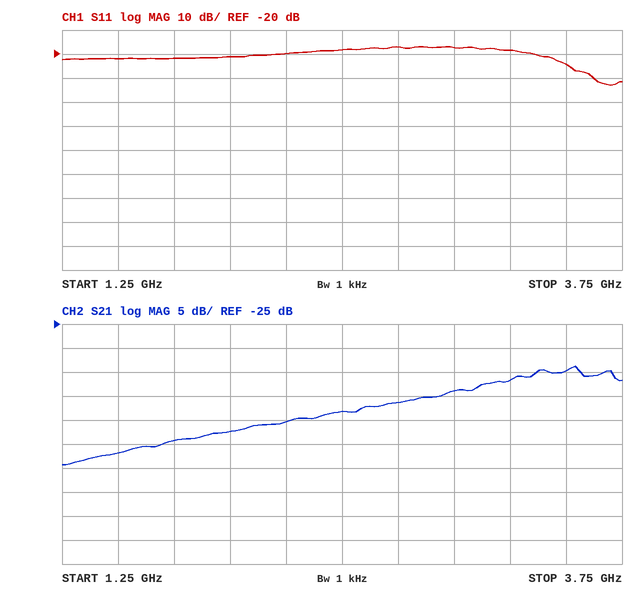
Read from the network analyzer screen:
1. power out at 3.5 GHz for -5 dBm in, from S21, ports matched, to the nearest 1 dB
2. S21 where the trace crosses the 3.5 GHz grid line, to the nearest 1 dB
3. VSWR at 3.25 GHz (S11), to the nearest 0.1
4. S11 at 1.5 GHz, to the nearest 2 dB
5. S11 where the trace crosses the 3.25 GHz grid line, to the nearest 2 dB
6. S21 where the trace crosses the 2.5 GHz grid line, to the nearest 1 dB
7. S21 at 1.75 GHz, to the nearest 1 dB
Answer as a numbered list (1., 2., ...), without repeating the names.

1. -40 dBm
2. -35 dB
3. 1.3
4. -22 dB
5. -18 dB
6. -43 dB
7. -49 dB
